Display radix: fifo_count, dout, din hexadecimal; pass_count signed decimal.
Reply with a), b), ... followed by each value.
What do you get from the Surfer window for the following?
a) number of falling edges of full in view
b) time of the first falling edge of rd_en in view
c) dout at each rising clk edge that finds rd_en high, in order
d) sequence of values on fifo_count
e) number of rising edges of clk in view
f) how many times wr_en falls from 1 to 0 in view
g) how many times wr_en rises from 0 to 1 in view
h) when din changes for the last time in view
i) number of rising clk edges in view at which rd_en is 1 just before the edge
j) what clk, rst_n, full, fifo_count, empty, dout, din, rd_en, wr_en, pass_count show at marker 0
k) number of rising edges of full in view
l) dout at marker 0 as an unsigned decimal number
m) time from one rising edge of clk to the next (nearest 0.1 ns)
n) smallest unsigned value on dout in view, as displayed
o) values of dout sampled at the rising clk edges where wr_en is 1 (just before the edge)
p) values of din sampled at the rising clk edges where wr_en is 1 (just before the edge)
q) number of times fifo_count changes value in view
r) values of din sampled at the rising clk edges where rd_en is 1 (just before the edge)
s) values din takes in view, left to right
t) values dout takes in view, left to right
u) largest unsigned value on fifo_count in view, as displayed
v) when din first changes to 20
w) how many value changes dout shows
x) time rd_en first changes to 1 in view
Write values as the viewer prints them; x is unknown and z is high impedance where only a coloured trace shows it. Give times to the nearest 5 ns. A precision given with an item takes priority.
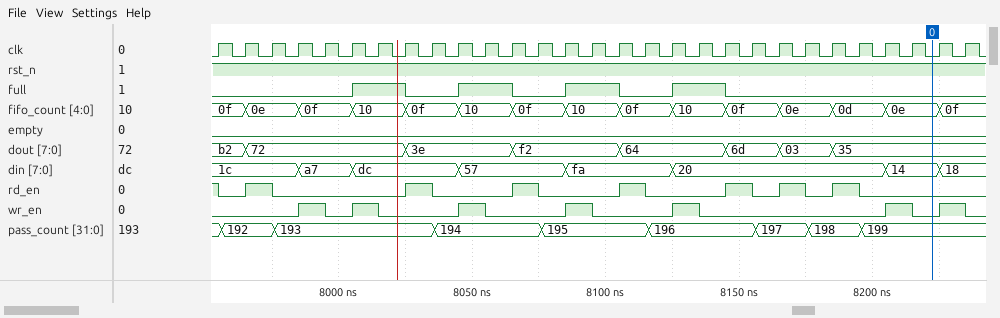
a) 4
b) 7955 ns
c) b2, 72, 3e, f2, 64, 6d, 03, 35
d) 0f, 0e, 0f, 10, 0f, 10, 0f, 10, 0f, 10, 0f, 0e, 0d, 0e, 0f
e) 29
f) 7
g) 7
h) 8225 ns
i) 8
j) clk=0, rst_n=1, full=0, fifo_count=0e, empty=0, dout=35, din=14, rd_en=0, wr_en=0, pass_count=199
k) 4
l) 53
m) 10 ns
n) 03
o) 72, 72, 3e, f2, 64, 35, 35
p) a7, dc, 57, fa, 20, 14, 18
q) 14
r) 1c, 1c, dc, 57, fa, 20, 20, 20
s) 1c, a7, dc, 57, fa, 20, 14, 18
t) b2, 72, 3e, f2, 64, 6d, 03, 35
u) 10
v) 8125 ns
w) 7
x) 7965 ns
